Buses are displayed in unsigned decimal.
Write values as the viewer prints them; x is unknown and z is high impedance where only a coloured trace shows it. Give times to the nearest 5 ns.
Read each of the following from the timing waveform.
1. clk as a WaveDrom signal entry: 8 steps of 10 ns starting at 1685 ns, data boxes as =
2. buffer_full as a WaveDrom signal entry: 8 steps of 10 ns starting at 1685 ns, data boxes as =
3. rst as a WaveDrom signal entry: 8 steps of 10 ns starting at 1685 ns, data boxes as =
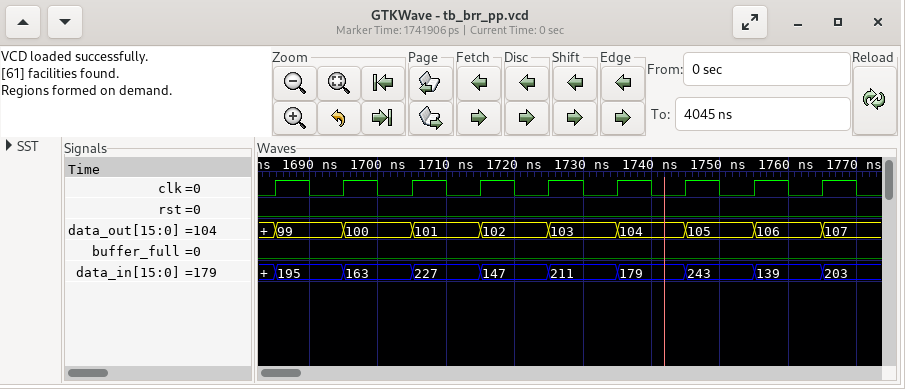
{name: 'clk', wave: 'p.......'}
{name: 'buffer_full', wave: '0.......'}
{name: 'rst', wave: '0.......'}
